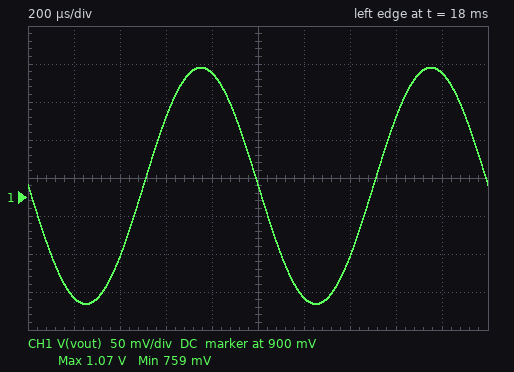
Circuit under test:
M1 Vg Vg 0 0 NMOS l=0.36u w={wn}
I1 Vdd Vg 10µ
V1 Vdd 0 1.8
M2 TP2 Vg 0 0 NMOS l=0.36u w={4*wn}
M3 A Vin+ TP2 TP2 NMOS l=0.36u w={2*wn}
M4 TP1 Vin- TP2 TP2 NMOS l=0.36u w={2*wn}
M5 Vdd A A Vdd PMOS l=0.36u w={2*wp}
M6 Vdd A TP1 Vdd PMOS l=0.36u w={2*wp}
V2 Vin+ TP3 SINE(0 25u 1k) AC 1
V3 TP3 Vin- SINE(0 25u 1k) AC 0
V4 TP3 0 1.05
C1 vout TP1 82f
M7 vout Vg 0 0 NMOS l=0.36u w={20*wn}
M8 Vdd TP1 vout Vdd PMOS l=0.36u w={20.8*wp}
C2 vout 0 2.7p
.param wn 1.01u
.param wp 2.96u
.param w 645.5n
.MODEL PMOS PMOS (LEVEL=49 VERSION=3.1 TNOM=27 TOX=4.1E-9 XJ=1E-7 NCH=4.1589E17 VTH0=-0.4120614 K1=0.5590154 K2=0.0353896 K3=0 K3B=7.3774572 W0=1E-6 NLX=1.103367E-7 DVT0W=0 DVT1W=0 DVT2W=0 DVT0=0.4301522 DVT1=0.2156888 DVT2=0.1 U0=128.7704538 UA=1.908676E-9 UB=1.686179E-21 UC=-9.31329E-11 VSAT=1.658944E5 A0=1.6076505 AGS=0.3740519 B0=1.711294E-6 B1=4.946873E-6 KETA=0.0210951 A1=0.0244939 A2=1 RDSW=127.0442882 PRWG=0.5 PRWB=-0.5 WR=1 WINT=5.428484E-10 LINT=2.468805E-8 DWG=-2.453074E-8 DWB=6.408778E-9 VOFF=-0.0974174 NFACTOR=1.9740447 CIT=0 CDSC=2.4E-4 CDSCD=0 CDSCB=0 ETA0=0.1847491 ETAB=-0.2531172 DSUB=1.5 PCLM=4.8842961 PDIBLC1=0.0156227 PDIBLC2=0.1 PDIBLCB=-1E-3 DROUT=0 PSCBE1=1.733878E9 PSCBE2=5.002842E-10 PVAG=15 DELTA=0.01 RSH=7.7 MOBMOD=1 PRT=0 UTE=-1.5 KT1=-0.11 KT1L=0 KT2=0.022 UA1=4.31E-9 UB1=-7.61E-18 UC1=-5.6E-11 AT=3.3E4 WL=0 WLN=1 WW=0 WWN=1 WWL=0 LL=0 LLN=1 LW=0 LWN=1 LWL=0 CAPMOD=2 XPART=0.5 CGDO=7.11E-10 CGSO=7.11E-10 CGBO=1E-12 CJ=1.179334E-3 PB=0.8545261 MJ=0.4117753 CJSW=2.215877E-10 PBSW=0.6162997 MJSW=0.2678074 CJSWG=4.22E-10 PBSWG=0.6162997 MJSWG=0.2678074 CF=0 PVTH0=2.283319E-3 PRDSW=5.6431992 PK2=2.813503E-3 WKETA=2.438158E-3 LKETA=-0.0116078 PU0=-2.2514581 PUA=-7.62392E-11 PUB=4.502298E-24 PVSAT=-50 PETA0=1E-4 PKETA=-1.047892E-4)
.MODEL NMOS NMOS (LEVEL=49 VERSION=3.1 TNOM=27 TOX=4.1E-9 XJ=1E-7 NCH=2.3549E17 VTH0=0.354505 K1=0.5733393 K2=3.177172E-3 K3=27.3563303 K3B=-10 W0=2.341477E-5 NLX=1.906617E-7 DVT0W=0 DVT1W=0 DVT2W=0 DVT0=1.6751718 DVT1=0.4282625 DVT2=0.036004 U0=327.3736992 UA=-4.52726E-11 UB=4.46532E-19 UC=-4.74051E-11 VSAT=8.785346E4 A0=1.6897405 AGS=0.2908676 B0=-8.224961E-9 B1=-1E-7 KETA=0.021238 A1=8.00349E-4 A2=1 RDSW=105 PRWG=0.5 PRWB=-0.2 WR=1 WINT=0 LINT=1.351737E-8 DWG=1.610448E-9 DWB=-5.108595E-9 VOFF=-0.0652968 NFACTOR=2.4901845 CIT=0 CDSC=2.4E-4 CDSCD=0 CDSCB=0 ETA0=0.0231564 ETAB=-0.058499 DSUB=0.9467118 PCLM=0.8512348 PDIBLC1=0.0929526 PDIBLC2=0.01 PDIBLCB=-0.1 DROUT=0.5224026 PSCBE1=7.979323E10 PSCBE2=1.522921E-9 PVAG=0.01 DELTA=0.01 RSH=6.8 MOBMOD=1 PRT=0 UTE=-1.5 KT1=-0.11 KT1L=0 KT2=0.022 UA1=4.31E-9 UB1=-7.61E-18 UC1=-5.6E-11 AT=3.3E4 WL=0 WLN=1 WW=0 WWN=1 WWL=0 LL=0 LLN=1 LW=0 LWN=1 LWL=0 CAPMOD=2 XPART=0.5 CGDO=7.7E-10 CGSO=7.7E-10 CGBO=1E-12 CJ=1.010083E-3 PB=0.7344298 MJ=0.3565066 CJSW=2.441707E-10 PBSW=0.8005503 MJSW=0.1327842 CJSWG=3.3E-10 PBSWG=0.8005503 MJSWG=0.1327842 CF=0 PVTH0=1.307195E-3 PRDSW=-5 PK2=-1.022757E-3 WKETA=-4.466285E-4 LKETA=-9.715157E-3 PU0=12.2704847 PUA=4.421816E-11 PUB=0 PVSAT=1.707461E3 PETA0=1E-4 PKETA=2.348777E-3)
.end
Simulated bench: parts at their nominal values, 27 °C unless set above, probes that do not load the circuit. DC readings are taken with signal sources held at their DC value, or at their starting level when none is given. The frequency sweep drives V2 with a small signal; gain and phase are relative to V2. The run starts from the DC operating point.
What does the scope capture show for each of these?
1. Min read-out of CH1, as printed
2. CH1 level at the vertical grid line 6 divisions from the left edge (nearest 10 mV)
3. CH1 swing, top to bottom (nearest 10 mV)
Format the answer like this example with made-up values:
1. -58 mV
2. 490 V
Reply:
1. 759 mV
2. 770 mV
3. 310 mV
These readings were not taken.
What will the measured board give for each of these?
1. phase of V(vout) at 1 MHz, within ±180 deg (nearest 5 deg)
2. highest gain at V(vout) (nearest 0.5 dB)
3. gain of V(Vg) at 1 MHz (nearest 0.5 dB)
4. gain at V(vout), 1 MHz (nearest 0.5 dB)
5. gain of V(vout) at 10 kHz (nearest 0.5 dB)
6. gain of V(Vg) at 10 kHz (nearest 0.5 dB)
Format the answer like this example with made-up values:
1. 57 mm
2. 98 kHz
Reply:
1. 95 deg
2. 70.0 dB
3. -13.5 dB
4. 48.5 dB
5. 70.0 dB
6. -32.5 dB
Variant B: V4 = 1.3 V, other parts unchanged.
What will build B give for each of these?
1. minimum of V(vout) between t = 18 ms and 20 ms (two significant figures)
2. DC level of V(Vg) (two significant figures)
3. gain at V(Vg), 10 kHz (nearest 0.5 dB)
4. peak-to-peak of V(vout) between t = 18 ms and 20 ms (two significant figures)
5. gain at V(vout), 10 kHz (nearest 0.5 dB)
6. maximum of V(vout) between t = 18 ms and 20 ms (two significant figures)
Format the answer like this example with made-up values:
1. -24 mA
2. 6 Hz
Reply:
1. 950 mV
2. 650 mV
3. -33.5 dB
4. 280 mV
5. 69.0 dB
6. 1.2 V
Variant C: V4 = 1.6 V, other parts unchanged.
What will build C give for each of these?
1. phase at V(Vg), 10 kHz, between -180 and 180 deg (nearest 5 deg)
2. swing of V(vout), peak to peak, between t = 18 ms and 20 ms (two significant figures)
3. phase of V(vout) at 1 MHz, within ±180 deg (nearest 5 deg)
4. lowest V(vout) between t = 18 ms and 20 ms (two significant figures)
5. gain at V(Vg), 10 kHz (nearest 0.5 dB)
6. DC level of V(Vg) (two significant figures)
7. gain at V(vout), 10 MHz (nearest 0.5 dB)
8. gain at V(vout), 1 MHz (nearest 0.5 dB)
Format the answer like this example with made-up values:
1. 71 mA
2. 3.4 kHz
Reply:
1. -90 deg
2. 90 mV
3. 105 deg
4. 1.2 V
5. -43.0 dB
6. 650 mV
7. 27.5 dB
8. 47.5 dB
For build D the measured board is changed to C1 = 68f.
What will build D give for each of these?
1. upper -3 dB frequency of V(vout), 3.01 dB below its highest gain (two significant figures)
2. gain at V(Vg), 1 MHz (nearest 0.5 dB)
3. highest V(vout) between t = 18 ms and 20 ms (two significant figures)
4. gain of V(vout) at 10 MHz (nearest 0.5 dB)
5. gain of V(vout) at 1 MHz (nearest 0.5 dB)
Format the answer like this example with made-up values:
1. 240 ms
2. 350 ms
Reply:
1. 98 kHz
2. -12.5 dB
3. 1.1 V
4. 29.5 dB
5. 49.5 dB
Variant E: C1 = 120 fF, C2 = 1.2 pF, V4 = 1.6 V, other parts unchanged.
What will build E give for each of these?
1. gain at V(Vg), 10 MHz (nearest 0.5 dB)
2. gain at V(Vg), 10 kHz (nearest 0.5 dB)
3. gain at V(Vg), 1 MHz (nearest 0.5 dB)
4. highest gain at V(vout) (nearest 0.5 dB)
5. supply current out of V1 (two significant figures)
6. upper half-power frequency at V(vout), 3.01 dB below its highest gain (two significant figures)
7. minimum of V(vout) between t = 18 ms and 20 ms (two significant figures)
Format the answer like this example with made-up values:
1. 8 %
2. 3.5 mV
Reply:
1. -16.0 dB
2. -43.0 dB
3. -16.5 dB
4. 59.0 dB
5. 260 µA
6. 220 kHz
7. 1.2 V
